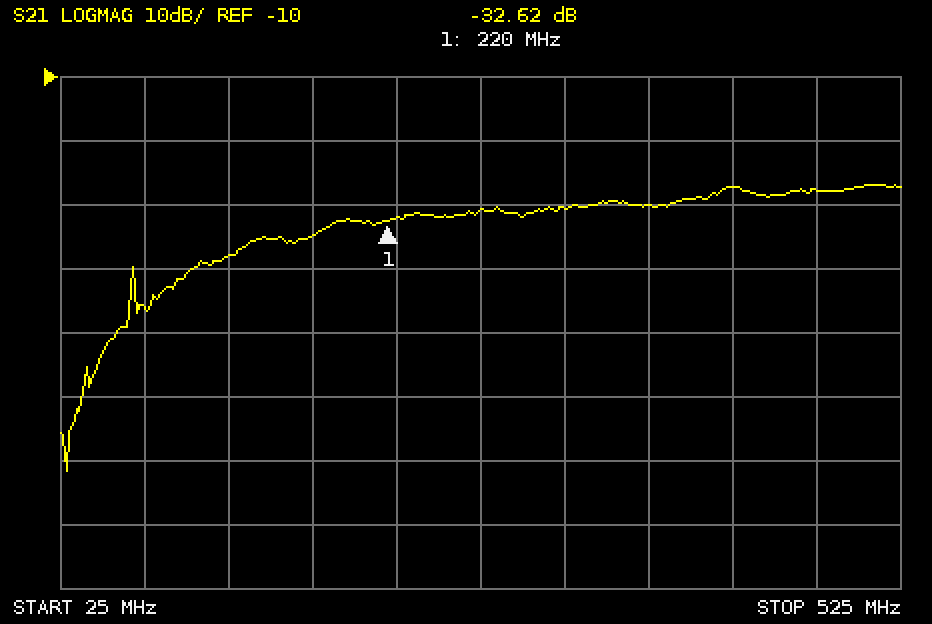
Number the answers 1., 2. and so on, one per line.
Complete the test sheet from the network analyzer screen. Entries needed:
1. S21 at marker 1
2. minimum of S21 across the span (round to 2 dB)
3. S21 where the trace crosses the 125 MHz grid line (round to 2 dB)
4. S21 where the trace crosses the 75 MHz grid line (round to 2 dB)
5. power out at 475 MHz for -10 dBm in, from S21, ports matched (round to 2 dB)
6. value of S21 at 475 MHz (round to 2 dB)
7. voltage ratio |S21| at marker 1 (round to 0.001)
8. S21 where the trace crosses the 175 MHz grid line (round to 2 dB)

1. -32.62 dB
2. -72 dB
3. -38 dB
4. -46 dB
5. -38 dBm
6. -28 dB
7. 0.023
8. -34 dB
